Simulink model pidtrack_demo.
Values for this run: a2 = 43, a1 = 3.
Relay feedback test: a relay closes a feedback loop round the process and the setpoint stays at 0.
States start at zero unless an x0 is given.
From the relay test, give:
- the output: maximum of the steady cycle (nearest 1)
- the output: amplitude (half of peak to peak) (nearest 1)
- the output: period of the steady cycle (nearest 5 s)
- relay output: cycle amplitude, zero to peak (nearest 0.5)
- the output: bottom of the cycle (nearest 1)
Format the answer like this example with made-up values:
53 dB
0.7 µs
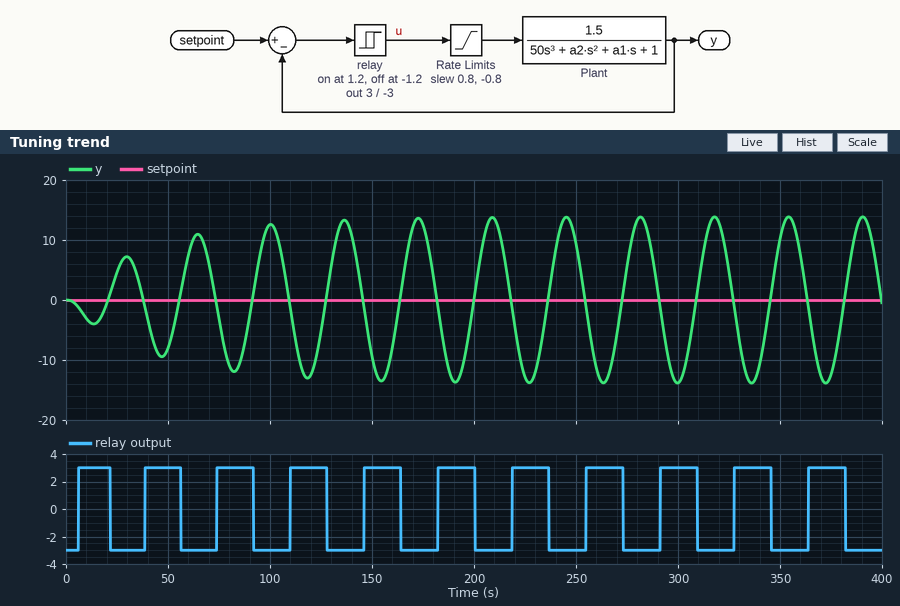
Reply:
14
14
35 s
3.0
-14
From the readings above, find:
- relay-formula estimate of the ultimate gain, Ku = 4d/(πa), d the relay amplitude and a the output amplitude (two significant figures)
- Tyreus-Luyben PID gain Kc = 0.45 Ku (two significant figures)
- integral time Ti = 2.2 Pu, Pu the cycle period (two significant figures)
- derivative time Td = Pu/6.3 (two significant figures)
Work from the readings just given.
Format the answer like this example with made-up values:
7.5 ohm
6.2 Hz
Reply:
0.27
0.12
77 s
5.6 s
